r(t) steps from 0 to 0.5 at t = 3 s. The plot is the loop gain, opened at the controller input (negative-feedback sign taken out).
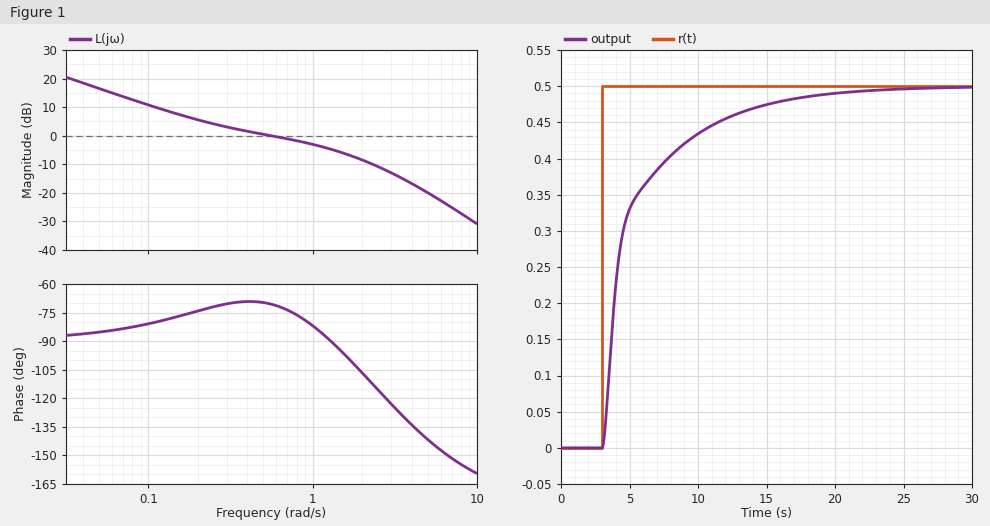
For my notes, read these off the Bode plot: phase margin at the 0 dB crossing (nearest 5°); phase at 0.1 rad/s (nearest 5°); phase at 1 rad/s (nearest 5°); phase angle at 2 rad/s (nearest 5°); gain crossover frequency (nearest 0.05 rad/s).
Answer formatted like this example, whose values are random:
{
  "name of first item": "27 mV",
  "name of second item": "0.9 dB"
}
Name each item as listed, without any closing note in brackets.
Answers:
{
  "phase margin at the 0 dB crossing": "110°",
  "phase at 0.1 rad/s": "-80°",
  "phase at 1 rad/s": "-80°",
  "phase angle at 2 rad/s": "-105°",
  "gain crossover frequency": "0.55 rad/s"
}
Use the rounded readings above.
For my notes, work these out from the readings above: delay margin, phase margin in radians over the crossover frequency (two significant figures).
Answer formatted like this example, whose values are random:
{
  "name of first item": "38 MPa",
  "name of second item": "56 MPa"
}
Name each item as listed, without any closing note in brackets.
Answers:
{
  "delay margin, phase margin in radians over the crossover frequency": "3.5 s"
}
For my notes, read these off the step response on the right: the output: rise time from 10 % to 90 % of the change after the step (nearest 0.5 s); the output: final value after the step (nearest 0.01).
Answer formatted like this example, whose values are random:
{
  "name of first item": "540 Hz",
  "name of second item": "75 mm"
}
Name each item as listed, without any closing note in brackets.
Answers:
{
  "the output: rise time from 10 % to 90 % of the change after the step": "8.0 s",
  "the output: final value after the step": "0.50"
}
